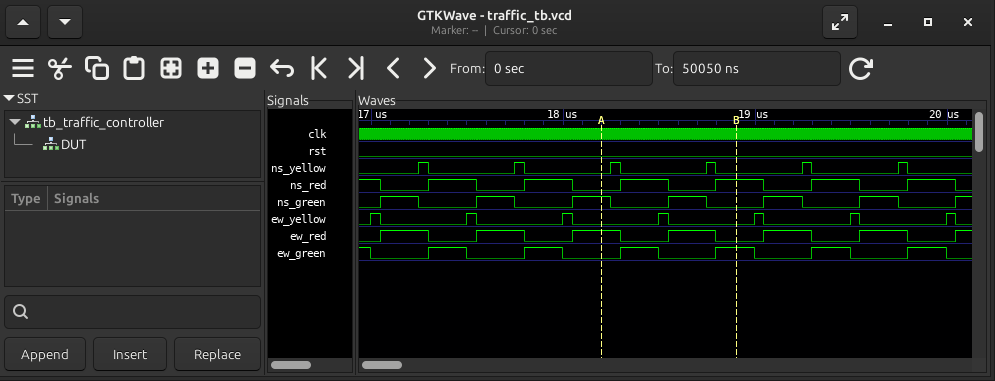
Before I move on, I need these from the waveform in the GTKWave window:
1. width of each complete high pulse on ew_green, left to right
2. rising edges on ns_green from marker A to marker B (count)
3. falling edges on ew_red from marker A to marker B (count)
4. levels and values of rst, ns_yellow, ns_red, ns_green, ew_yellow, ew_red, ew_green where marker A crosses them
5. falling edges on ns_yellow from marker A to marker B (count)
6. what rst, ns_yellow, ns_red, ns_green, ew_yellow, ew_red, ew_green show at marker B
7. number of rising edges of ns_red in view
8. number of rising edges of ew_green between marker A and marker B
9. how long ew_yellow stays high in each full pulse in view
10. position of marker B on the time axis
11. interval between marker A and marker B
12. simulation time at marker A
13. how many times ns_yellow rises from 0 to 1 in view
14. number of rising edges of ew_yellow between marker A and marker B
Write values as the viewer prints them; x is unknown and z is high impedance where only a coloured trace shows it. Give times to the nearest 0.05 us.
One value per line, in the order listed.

0.2 us, 0.2 us, 0.2 us, 0.2 us, 0.2 us, 0.2 us
1
2
rst=0, ns_yellow=0, ns_red=0, ns_green=1, ew_yellow=0, ew_red=1, ew_green=0
2
rst=0, ns_yellow=0, ns_red=1, ns_green=0, ew_yellow=0, ew_red=0, ew_green=1
6
2
0.05 us, 0.05 us, 0.05 us, 0.05 us, 0.05 us, 0.05 us, 0.05 us
18.9 us
0.7 us
18.2 us
6
1
